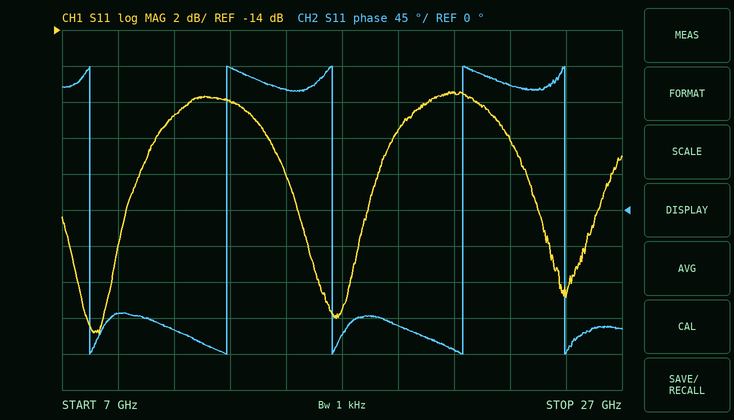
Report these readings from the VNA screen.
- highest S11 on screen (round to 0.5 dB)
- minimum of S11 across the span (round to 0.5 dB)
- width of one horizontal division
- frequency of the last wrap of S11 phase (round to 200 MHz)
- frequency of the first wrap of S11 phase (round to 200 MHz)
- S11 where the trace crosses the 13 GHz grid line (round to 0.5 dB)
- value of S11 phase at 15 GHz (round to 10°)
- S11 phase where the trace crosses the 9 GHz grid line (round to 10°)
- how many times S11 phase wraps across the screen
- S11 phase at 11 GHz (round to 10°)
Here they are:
-17.5 dB
-31.0 dB
2 GHz
25.0 GHz
8.0 GHz
-18.0 dB
150°
-130°
5
-150°
